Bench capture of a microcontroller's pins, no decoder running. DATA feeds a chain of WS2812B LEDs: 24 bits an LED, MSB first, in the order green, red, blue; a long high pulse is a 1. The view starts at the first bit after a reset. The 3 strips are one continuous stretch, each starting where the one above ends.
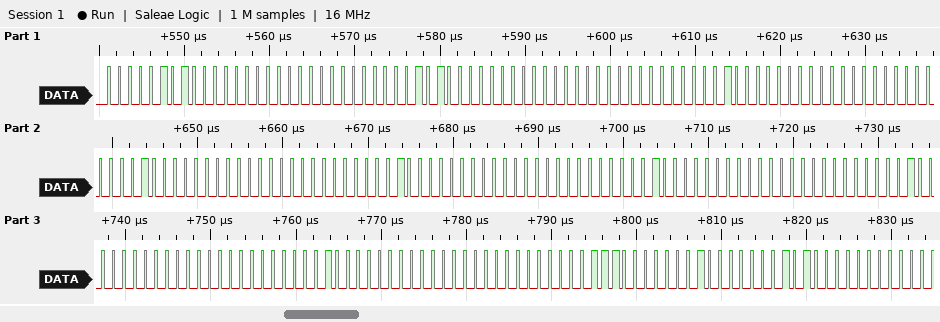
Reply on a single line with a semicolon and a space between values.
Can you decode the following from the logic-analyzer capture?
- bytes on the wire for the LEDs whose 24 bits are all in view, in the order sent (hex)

05 00 00 05 00 00 00 20 00 00 20 00 00 20 00 00 20 00 00 20 00 00 20 00 00 1C 04
